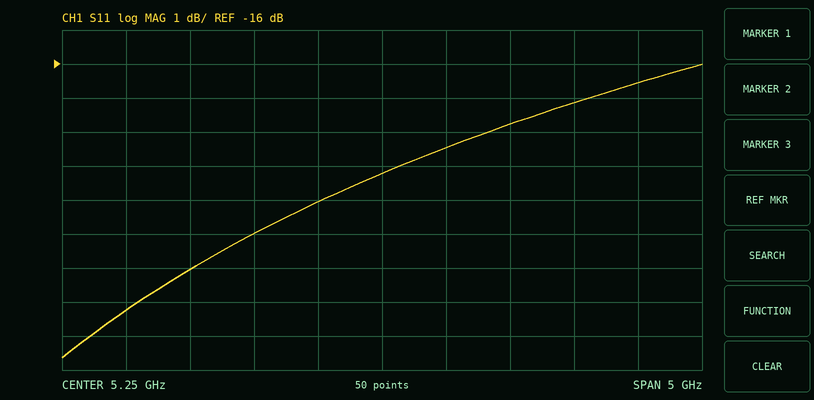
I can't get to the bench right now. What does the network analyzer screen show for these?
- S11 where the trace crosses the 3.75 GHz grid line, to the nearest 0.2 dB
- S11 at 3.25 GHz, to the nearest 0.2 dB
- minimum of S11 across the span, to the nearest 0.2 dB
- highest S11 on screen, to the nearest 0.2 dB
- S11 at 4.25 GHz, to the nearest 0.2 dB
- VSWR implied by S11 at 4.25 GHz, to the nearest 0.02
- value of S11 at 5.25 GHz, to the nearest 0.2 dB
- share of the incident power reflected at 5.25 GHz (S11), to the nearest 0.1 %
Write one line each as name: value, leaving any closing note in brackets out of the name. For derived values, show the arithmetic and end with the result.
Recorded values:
S11 where the trace crosses the 3.75 GHz grid line, to the nearest 0.2 dB: -22.0 dB
S11 at 3.25 GHz, to the nearest 0.2 dB: -23.2 dB
minimum of S11 across the span, to the nearest 0.2 dB: -24.6 dB
highest S11 on screen, to the nearest 0.2 dB: -16.0 dB
S11 at 4.25 GHz, to the nearest 0.2 dB: -21.0 dB
VSWR implied by S11 at 4.25 GHz, to the nearest 0.02: |Γ| = 10^(-21/20) = 0.0891; VSWR = (1 + 0.0891)/(1 − 0.0891) ≈ 1.20
value of S11 at 5.25 GHz, to the nearest 0.2 dB: -19.2 dB
share of the incident power reflected at 5.25 GHz (S11), to the nearest 0.1 %: 10^(-19.2/10) ≈ 1.2 %
